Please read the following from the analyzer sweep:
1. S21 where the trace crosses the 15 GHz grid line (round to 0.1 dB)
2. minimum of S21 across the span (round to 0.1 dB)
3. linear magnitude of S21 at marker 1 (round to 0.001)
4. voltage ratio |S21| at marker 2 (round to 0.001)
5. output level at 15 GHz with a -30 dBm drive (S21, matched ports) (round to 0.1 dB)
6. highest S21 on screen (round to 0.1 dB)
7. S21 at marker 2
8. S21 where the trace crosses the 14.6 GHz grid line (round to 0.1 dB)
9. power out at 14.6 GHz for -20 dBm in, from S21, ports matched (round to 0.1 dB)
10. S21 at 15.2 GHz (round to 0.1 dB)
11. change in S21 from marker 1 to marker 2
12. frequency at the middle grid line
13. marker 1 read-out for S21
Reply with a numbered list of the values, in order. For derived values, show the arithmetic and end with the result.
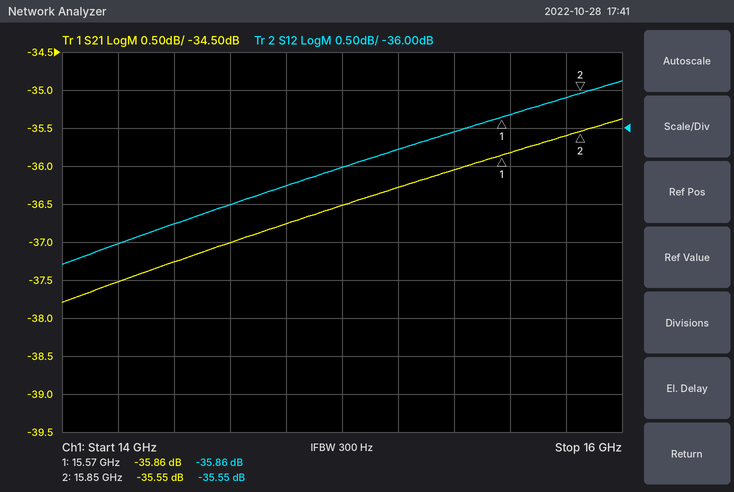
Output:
1. -36.5 dB
2. -37.8 dB
3. 10^(-35.86/20) ≈ 0.016
4. 10^(-35.55/20) ≈ 0.017
5. -30 dBm + (-36.5 dB) = -66.5 dBm
6. -35.4 dB
7. -35.55 dB
8. -37.0 dB
9. -20 dBm + (-37.0 dB) = -57.0 dBm
10. -36.3 dB
11. -35.55 − (-35.86) = 0.31 dB
12. 15 GHz
13. -35.86 dB
